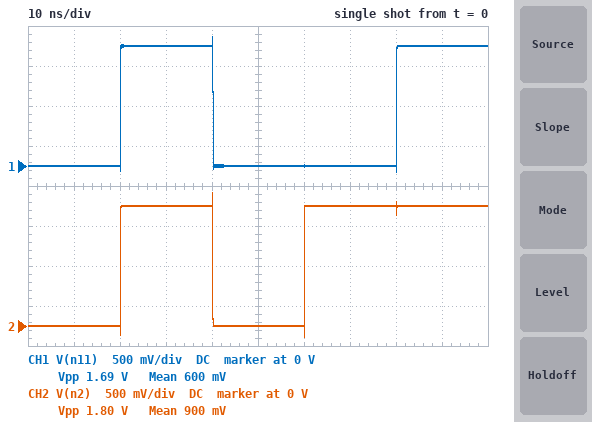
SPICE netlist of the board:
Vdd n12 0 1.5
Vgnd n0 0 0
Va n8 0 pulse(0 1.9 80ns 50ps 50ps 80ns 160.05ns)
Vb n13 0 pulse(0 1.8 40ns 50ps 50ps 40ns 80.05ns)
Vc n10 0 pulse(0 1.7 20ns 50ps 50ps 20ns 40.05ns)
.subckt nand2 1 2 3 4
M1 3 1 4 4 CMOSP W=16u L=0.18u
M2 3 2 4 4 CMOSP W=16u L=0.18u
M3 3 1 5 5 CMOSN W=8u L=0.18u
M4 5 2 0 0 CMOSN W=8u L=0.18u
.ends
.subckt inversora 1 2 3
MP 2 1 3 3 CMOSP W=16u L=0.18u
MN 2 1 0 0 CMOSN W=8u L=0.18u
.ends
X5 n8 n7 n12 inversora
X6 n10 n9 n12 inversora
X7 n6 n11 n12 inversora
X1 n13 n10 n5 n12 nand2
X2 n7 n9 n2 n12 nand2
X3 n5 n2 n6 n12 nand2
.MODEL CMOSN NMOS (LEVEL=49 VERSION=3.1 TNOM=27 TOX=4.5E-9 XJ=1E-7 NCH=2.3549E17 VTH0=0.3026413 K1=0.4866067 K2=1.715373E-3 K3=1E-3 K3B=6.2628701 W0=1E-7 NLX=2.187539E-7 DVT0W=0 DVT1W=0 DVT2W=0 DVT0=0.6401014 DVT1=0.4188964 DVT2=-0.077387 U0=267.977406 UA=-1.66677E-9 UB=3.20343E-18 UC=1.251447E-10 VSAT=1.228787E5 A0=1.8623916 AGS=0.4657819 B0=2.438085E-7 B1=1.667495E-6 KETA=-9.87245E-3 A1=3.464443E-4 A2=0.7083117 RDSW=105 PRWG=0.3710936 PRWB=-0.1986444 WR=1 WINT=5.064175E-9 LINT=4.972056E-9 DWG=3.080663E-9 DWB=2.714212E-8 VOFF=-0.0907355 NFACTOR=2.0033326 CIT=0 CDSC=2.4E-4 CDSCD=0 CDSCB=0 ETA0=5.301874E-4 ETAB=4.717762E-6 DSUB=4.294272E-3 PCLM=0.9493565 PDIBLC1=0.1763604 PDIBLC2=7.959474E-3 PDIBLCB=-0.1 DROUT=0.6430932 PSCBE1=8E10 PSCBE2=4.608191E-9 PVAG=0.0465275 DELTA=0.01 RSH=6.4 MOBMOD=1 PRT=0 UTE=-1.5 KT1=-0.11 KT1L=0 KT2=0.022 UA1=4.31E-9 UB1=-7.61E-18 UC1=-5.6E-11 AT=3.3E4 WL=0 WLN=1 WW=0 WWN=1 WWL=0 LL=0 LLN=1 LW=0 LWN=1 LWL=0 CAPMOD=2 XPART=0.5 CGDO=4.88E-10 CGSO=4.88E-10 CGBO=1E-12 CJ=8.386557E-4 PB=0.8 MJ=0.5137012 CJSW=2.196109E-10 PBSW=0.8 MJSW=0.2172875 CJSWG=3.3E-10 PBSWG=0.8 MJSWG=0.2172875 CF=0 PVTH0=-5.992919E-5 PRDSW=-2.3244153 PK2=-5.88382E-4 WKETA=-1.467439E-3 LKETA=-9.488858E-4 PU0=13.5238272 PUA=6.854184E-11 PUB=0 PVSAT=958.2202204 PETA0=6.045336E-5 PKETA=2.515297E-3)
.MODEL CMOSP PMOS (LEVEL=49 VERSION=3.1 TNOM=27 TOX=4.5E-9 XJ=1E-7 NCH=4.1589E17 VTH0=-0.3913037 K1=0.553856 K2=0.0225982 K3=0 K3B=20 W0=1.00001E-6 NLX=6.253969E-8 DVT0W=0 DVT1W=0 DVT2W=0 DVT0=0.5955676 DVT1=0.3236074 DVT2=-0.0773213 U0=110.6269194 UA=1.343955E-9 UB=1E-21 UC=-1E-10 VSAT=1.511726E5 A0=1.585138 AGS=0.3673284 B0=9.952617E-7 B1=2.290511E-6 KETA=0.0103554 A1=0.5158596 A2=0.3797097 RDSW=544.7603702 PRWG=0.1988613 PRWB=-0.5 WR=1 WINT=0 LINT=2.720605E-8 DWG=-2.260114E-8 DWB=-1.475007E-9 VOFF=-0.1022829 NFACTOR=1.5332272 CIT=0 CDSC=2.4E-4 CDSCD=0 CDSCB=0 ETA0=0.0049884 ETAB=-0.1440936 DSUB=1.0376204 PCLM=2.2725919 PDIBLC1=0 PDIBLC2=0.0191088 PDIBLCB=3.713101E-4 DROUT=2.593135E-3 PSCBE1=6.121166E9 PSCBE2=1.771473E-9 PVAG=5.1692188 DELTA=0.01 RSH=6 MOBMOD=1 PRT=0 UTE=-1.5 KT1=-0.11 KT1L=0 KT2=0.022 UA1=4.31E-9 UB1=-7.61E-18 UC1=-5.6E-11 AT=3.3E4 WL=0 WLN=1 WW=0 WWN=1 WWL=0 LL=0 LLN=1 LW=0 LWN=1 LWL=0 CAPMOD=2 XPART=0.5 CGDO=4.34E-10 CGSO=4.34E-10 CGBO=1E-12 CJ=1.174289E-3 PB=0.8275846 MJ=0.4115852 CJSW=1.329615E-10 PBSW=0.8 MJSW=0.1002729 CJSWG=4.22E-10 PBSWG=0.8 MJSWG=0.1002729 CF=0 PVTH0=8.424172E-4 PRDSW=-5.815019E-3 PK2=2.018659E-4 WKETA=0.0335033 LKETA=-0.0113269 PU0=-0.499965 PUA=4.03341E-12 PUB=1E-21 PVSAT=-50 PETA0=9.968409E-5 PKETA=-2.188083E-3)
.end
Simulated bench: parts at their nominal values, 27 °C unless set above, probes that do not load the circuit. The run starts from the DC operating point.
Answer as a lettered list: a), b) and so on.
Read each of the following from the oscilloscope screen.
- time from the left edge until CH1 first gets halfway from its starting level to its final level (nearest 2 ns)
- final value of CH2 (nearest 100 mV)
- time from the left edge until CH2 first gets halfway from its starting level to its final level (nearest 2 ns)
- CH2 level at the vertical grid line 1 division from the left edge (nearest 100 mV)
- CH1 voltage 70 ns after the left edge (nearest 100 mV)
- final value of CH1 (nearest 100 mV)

a) 20 ns
b) 1.5 V
c) 20 ns
d) 0 V
e) 0 V
f) 1.5 V
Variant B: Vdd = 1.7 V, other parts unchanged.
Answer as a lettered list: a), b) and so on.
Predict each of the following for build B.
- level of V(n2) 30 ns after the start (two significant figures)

a) 1.7 V
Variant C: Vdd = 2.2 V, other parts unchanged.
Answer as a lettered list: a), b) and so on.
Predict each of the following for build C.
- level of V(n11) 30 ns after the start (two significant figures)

a) 2.2 V
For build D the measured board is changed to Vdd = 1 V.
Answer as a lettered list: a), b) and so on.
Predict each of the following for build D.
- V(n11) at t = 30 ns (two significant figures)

a) 1.0 V
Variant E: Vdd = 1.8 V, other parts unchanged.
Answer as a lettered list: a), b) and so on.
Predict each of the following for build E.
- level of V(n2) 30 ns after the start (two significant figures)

a) 1.8 V
